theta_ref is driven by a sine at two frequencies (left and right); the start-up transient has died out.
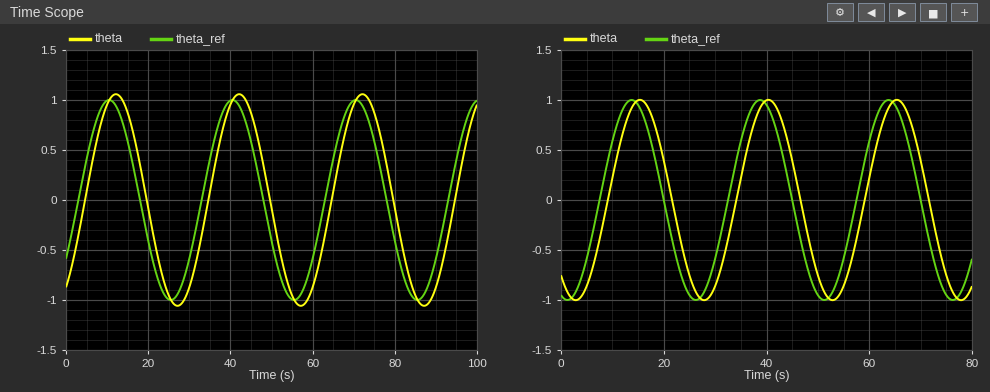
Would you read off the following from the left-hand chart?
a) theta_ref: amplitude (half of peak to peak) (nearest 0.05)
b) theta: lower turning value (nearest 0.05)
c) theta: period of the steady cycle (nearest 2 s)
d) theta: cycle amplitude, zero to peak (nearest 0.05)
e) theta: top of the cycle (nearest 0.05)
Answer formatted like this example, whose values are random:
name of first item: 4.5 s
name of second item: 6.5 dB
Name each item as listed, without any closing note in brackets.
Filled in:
theta_ref: amplitude (half of peak to peak): 1.00
theta: lower turning value: -1.05
theta: period of the steady cycle: 30 s
theta: cycle amplitude, zero to peak: 1.05
theta: top of the cycle: 1.05
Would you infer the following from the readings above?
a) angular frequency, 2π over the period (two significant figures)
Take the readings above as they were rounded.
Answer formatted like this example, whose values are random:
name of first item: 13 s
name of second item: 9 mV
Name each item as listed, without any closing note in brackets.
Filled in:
angular frequency, 2π over the period: 0.21 rad/s
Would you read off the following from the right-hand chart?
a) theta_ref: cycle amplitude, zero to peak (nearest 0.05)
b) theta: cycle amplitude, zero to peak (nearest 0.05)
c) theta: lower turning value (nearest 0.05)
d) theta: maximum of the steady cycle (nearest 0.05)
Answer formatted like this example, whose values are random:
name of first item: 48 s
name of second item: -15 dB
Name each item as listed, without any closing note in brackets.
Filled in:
theta_ref: cycle amplitude, zero to peak: 1.00
theta: cycle amplitude, zero to peak: 1.00
theta: lower turning value: -1.00
theta: maximum of the steady cycle: 1.00
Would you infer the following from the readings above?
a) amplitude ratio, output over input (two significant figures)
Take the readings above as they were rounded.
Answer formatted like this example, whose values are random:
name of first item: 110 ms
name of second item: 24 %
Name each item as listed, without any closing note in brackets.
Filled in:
amplitude ratio, output over input: 1.0
